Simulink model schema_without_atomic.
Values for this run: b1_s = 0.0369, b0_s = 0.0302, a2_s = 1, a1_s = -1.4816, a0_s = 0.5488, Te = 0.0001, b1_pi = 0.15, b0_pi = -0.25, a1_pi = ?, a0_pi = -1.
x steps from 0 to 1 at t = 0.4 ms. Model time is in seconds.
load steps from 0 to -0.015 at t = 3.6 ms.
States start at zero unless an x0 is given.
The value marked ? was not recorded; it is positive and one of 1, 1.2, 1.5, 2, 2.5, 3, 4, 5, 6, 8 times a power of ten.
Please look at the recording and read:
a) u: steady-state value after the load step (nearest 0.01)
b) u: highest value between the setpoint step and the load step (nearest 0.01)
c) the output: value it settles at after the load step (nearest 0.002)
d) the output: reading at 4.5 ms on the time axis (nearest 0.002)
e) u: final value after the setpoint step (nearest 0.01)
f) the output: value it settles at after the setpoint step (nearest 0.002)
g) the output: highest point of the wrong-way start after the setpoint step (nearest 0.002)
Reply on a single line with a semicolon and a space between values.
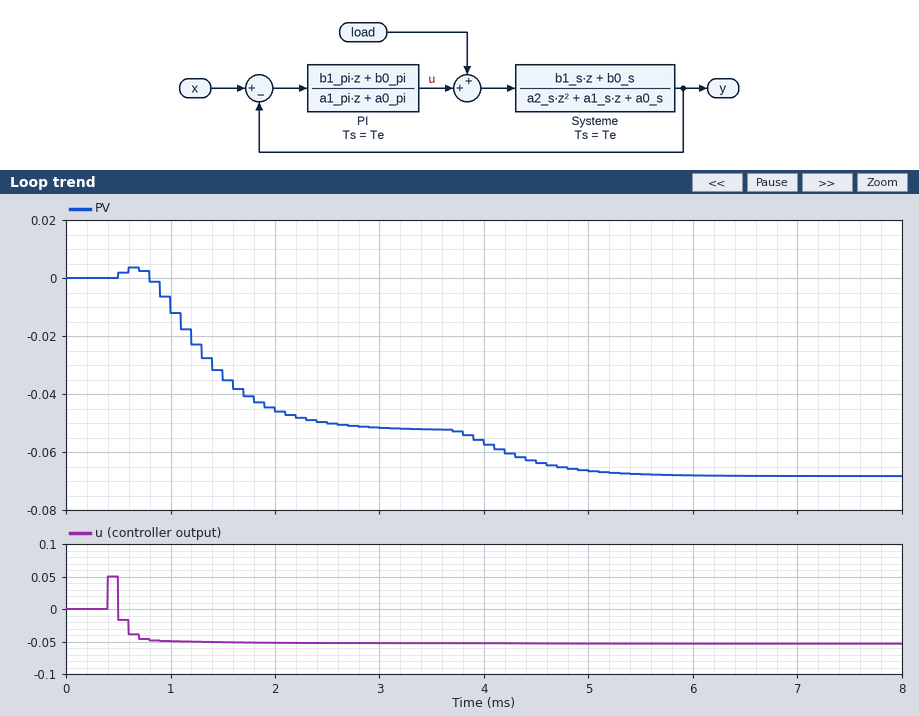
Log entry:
-0.05; 0.05; -0.068; -0.064; -0.05; -0.052; 0.004
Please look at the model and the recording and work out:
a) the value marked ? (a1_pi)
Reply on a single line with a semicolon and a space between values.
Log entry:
3
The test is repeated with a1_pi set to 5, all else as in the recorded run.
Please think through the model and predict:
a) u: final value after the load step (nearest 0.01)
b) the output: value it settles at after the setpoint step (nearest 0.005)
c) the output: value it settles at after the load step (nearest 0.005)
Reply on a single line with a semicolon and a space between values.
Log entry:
-0.03; -0.025; -0.040
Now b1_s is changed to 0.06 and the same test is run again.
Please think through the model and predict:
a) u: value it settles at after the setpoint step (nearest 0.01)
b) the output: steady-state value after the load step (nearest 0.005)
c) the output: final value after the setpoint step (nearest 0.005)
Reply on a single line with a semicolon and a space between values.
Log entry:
-0.05; -0.095; -0.070
